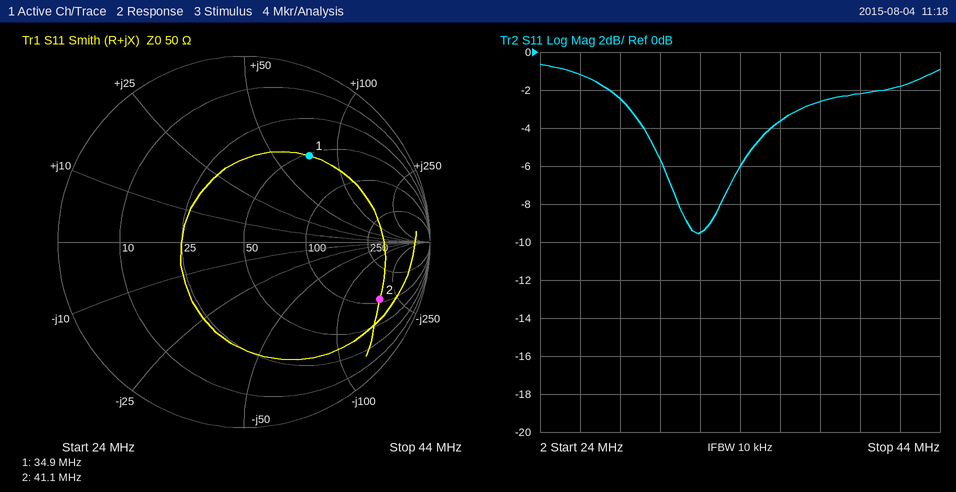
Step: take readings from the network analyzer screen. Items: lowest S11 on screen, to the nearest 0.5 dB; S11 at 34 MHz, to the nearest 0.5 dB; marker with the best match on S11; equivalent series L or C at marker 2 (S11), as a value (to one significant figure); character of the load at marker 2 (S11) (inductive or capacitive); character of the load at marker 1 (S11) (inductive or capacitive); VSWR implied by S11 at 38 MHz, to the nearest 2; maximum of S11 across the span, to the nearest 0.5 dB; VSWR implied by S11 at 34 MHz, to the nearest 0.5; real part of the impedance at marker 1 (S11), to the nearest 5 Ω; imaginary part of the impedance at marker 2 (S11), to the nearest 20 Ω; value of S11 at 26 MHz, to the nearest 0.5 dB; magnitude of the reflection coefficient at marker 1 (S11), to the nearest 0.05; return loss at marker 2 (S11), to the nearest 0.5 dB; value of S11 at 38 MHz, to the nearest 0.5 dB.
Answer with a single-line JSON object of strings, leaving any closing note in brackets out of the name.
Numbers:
{"lowest S11 on screen, to the nearest 0.5 dB": "-9.5 dB", "S11 at 34 MHz, to the nearest 0.5 dB": "-6.0 dB", "marker with the best match on S11": "marker 1", "equivalent series L or C at marker 2 (S11), as a value": "20 pF", "character of the load at marker 2 (S11)": "capacitive", "character of the load at marker 1 (S11)": "inductive", "VSWR implied by S11 at 38 MHz, to the nearest 2": "6", "maximum of S11 across the span, to the nearest 0.5 dB": "-0.5 dB", "VSWR implied by S11 at 34 MHz, to the nearest 0.5": "3.0", "real part of the impedance at marker 1 (S11), to the nearest 5 Ω": "50 Ω", "imaginary part of the impedance at marker 2 (S11), to the nearest 20 Ω": "-180 Ω", "value of S11 at 26 MHz, to the nearest 0.5 dB": "-1.0 dB", "magnitude of the reflection coefficient at marker 1 (S11), to the nearest 0.05": "0.60", "return loss at marker 2 (S11), to the nearest 0.5 dB": "2.0 dB", "value of S11 at 38 MHz, to the nearest 0.5 dB": "-2.5 dB"}
